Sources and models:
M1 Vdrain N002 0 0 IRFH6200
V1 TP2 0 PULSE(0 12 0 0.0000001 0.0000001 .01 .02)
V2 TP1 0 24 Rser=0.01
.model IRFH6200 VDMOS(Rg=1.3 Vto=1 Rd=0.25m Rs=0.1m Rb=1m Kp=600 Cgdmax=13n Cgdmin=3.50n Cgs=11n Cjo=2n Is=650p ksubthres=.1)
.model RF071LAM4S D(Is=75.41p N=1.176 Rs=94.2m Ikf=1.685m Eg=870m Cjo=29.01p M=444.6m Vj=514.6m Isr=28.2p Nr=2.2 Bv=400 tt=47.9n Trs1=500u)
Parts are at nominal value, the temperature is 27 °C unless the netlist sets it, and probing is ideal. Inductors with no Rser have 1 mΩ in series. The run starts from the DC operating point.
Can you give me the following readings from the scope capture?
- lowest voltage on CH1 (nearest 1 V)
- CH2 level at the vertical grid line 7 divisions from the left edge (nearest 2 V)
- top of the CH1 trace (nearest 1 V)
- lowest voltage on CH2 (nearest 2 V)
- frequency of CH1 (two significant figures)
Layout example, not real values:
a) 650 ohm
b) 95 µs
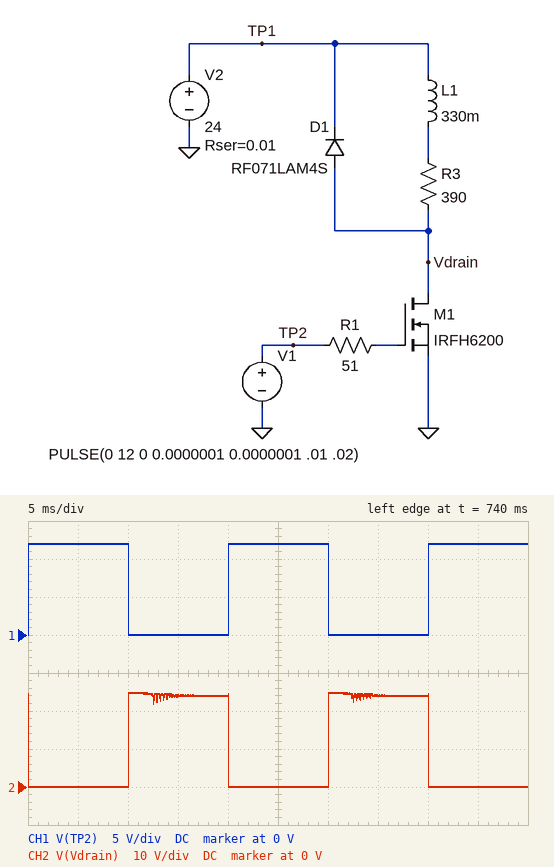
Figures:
a) 0 V
b) 24 V
c) 12 V
d) 0 V
e) 50 Hz
